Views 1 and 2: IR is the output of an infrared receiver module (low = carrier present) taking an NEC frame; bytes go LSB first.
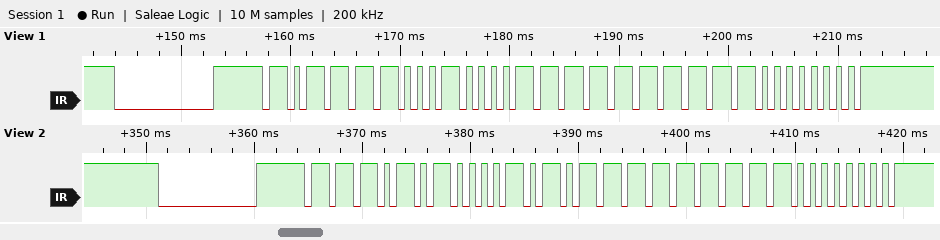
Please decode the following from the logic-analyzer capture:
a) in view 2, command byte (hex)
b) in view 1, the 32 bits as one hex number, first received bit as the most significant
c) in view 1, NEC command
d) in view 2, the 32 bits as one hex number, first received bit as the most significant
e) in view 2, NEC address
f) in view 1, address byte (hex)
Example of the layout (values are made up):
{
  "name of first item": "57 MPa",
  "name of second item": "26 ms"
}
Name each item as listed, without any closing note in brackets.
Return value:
{
  "in view 2, command byte": "0xFF",
  "in view 1, the 32 bits as one hex number, first received bit as the most significant": "0xBC43FF00",
  "in view 1, NEC command": "0xFF",
  "in view 2, the 32 bits as one hex number, first received bit as the most significant": "0xEA15FF00",
  "in view 2, NEC address": "0x57",
  "in view 1, address byte": "0x3D"
}
